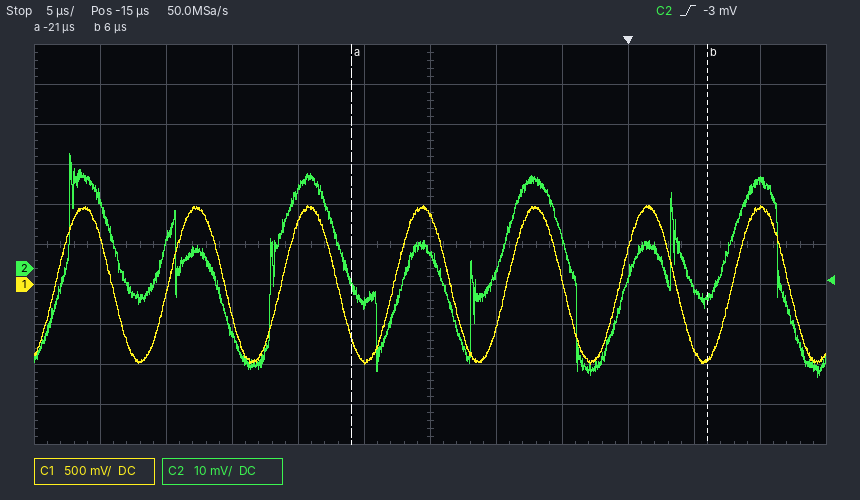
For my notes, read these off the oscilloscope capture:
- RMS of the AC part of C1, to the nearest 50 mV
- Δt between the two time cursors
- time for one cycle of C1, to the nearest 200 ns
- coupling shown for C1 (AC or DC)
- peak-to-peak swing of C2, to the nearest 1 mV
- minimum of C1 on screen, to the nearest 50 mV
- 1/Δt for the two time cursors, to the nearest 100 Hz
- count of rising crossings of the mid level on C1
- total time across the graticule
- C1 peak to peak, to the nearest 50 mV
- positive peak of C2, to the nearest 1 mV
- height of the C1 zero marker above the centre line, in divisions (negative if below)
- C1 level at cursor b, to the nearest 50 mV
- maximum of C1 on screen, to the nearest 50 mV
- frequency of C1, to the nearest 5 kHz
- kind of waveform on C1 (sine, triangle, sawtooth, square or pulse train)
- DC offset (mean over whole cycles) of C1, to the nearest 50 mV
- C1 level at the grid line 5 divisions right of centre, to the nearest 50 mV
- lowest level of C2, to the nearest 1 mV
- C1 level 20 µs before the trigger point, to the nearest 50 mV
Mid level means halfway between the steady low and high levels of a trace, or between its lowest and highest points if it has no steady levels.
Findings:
700 mV
27.0 µs
8.6 µs
DC
56 mV
-1.00 V
37.0 kHz
7
60 µs
2.00 V
29 mV
-1.0 div
-950 mV
1.00 V
115 kHz
sine
0 mV
950 mV
-27 mV
-950 mV
